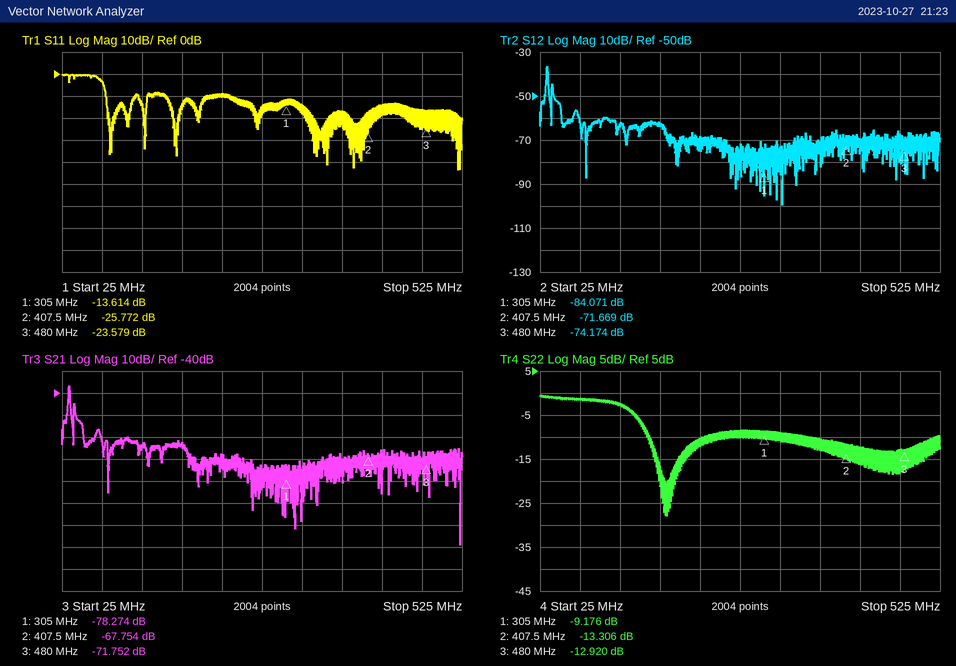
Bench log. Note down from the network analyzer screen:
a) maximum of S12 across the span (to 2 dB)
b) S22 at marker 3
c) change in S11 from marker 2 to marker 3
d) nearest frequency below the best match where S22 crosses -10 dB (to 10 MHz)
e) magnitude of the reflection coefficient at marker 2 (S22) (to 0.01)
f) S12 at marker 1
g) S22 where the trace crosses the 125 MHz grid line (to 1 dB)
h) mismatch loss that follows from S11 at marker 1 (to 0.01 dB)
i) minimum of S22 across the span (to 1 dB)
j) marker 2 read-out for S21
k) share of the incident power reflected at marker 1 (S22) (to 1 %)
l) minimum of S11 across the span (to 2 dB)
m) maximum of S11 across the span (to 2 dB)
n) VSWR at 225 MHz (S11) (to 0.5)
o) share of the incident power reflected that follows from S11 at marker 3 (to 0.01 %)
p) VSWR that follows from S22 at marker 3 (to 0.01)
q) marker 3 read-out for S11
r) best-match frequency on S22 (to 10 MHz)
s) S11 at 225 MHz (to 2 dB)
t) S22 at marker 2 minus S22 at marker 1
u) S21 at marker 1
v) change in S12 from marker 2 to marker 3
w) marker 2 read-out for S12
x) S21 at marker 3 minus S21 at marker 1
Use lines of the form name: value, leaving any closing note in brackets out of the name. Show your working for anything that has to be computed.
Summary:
maximum of S12 across the span: -36 dB
S22 at marker 3: -12.920 dB
change in S11 from marker 2 to marker 3: -23.579 − (-25.772) = 2.193 dB
nearest frequency below the best match where S22 crosses -10 dB: 160 MHz
magnitude of the reflection coefficient at marker 2 (S22): 10^(-13.306/20) ≈ 0.22
S12 at marker 1: -84.071 dB
S22 where the trace crosses the 125 MHz grid line: -3 dB
mismatch loss that follows from S11 at marker 1: −10 log10(1 − 10^(-13.614/10)) ≈ 0.19 dB
minimum of S22 across the span: -28 dB
marker 2 read-out for S21: -67.754 dB
share of the incident power reflected at marker 1 (S22): 10^(-9.176/10) ≈ 12 %
minimum of S11 across the span: -44 dB
maximum of S11 across the span: 0 dB
VSWR at 225 MHz (S11): |Γ| = 10^(-10/20) = 0.3162; VSWR = (1 + 0.3162)/(1 − 0.3162) ≈ 1.92, so 2.0 to the nearest 0.5
share of the incident power reflected that follows from S11 at marker 3: 10^(-23.579/10) ≈ 0.44 %
VSWR that follows from S22 at marker 3: (1 + 0.2259)/(1 − 0.2259) ≈ 1.58
marker 3 read-out for S11: -23.579 dB
best-match frequency on S22: 180 MHz
S11 at 225 MHz: -10 dB
S22 at marker 2 minus S22 at marker 1: -13.306 − (-9.176) = -4.130 dB
S21 at marker 1: -78.274 dB
change in S12 from marker 2 to marker 3: -74.174 − (-71.669) = -2.505 dB
marker 2 read-out for S12: -71.669 dB
S21 at marker 3 minus S21 at marker 1: -71.752 − (-78.274) = 6.522 dB
